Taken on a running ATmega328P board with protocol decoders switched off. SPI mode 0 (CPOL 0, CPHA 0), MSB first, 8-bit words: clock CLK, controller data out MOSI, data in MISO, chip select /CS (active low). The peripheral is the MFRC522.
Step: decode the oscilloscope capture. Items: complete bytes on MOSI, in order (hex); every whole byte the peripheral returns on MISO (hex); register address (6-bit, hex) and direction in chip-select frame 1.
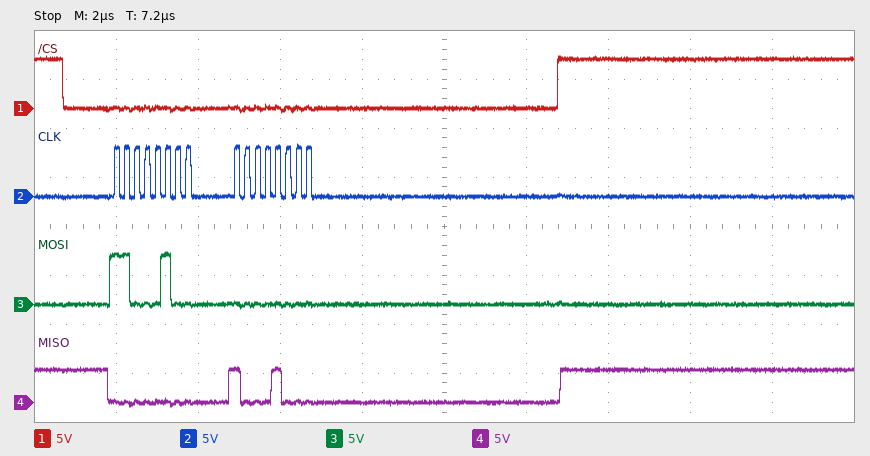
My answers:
C4 00
00 88
0x22 read
